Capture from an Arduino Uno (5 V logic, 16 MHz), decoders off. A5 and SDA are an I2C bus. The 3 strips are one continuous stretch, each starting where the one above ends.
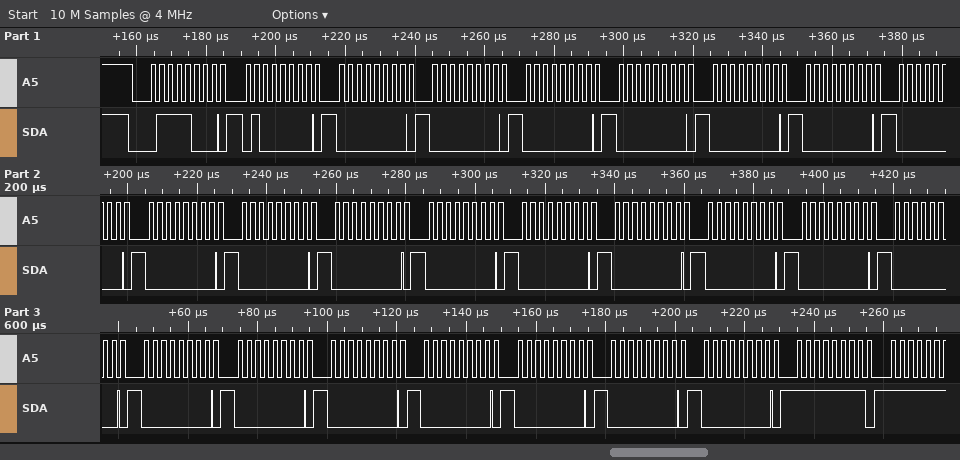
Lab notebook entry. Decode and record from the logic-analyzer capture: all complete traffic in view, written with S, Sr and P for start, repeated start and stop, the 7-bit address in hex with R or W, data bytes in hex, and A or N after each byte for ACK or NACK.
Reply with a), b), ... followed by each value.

a) S 3CW A 40 A 00 A 00 A 00 A 00 A 00 A 00 A 00 A 00 A 00 A 00 A 00 A 00 A 00 A 00 A 00 A 00 A 00 A 00 A 00 A 00 A 00 A 00 A 00 A FF A
